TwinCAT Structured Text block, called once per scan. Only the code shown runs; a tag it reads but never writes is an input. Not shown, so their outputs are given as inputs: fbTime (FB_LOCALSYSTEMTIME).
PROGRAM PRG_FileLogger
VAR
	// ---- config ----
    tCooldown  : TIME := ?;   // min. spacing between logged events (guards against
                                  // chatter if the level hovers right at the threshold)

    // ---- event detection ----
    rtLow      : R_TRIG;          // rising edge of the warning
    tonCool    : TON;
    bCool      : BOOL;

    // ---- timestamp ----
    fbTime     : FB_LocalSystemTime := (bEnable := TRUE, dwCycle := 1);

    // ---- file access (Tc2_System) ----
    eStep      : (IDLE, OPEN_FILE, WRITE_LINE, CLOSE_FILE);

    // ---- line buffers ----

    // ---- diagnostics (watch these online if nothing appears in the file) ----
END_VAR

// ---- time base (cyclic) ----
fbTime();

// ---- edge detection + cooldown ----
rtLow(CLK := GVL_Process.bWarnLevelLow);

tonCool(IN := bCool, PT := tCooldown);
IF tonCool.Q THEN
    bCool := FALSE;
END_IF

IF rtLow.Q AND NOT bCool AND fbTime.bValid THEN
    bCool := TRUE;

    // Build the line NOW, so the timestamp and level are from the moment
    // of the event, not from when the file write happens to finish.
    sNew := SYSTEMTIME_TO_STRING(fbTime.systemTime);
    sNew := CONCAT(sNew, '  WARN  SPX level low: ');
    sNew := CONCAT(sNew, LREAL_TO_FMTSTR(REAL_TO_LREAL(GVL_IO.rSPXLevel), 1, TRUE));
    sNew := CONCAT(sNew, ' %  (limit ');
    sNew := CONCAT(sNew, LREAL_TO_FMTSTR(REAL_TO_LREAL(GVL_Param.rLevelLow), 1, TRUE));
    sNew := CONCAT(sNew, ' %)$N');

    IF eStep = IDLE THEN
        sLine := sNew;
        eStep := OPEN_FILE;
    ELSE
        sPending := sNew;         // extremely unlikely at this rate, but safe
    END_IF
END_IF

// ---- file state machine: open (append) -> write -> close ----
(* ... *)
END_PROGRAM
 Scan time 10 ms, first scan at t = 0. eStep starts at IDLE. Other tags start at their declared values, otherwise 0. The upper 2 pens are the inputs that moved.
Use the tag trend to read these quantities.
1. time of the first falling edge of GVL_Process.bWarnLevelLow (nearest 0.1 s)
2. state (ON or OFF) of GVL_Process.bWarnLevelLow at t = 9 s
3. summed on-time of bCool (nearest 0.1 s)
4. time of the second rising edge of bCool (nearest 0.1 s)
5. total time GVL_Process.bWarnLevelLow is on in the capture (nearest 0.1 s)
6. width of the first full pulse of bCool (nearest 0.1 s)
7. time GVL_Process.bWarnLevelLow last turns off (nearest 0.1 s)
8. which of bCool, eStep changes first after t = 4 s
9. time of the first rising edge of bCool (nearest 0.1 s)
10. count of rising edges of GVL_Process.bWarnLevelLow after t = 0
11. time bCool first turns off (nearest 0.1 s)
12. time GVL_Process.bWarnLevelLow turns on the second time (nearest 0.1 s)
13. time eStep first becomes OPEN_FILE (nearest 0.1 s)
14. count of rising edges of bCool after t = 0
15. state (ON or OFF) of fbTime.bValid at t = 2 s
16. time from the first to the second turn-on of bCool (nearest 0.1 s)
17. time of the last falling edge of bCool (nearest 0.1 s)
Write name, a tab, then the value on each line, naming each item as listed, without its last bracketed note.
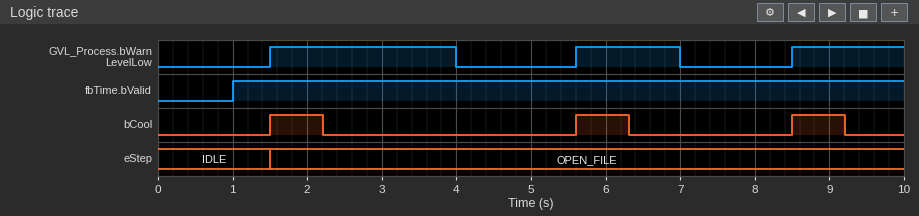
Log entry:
time of the first falling edge of GVL_Process.bWarnLevelLow	4.0 s
state (ON or OFF) of GVL_Process.bWarnLevelLow at t = 9 s	ON
summed on-time of bCool	2.1 s
time of the second rising edge of bCool	5.6 s
total time GVL_Process.bWarnLevelLow is on in the capture	5.4 s
width of the first full pulse of bCool	0.7 s
time GVL_Process.bWarnLevelLow last turns off	7.0 s
which of bCool, eStep changes first after t = 4 s	bCool
time of the first rising edge of bCool	1.5 s
count of rising edges of GVL_Process.bWarnLevelLow after t = 0	3
time bCool first turns off	2.2 s
time GVL_Process.bWarnLevelLow turns on the second time	5.6 s
time eStep first becomes OPEN_FILE	1.5 s
count of rising edges of bCool after t = 0	3
state (ON or OFF) of fbTime.bValid at t = 2 s	ON
time from the first to the second turn-on of bCool	4.1 s
time of the last falling edge of bCool	9.2 s
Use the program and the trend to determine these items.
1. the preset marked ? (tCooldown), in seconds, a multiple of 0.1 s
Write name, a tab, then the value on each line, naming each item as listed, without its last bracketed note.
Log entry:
the preset marked ? (tCooldown), in seconds, a multiple of 0.1 s	0.7 s
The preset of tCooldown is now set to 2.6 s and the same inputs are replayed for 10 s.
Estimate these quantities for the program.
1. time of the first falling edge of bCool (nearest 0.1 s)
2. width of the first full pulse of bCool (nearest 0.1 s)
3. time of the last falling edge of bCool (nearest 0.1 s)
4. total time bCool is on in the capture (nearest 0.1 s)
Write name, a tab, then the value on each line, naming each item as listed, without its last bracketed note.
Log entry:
time of the first falling edge of bCool	4.1 s
width of the first full pulse of bCool	2.6 s
time of the last falling edge of bCool	8.2 s
total time bCool is on in the capture	6.7 s
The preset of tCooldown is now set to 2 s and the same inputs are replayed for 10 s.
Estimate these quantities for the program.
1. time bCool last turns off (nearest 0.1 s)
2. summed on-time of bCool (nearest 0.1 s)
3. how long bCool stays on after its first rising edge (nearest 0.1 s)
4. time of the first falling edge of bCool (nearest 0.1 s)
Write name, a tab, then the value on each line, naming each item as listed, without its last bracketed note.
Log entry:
time bCool last turns off	7.6 s
summed on-time of bCool	5.5 s
how long bCool stays on after its first rising edge	2.0 s
time of the first falling edge of bCool	3.5 s
